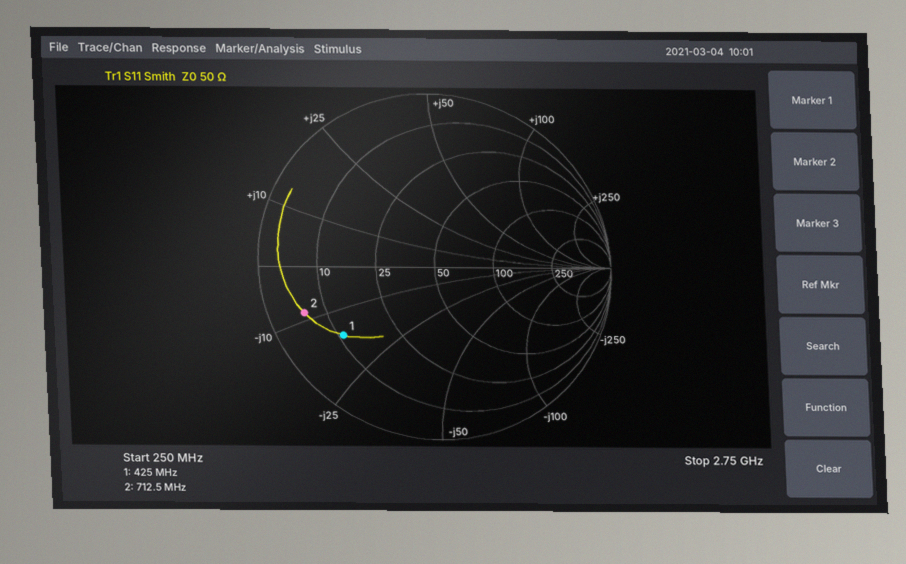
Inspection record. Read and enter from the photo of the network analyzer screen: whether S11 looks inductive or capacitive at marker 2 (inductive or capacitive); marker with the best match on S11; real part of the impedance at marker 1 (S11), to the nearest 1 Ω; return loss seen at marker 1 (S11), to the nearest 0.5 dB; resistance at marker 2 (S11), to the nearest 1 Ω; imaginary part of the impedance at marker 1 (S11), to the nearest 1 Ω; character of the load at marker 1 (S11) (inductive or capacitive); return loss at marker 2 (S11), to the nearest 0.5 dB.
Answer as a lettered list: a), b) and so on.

a) capacitive
b) marker 1
c) 11 Ω
d) 3.5 dB
e) 6 Ω
f) -16 Ω
g) capacitive
h) 2.0 dB
